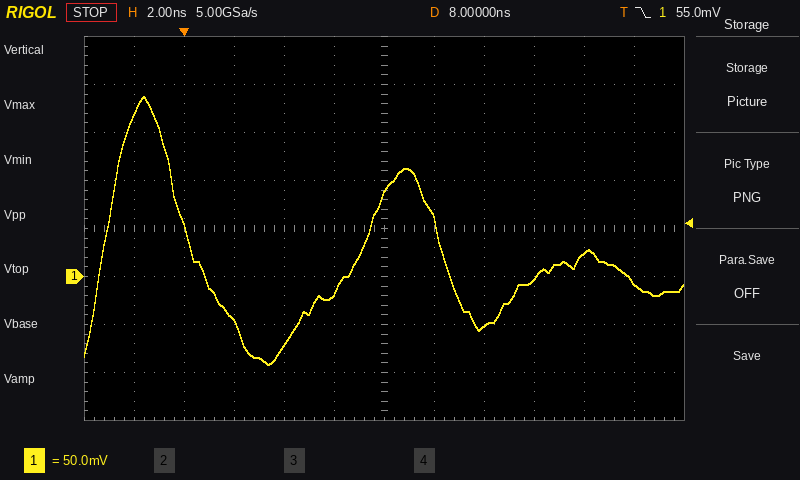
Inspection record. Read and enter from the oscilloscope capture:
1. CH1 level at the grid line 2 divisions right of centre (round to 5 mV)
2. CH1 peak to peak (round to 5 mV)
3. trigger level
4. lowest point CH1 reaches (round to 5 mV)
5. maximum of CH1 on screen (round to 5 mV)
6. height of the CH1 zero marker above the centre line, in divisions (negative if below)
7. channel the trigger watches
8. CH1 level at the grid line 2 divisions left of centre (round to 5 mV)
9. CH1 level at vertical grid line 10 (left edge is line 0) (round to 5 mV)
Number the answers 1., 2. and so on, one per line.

1. -50 mV
2. 280 mV
3. 55.0 mV
4. -90 mV
5. 190 mV
6. -1.0 div
7. CH1
8. -70 mV
9. 25 mV
